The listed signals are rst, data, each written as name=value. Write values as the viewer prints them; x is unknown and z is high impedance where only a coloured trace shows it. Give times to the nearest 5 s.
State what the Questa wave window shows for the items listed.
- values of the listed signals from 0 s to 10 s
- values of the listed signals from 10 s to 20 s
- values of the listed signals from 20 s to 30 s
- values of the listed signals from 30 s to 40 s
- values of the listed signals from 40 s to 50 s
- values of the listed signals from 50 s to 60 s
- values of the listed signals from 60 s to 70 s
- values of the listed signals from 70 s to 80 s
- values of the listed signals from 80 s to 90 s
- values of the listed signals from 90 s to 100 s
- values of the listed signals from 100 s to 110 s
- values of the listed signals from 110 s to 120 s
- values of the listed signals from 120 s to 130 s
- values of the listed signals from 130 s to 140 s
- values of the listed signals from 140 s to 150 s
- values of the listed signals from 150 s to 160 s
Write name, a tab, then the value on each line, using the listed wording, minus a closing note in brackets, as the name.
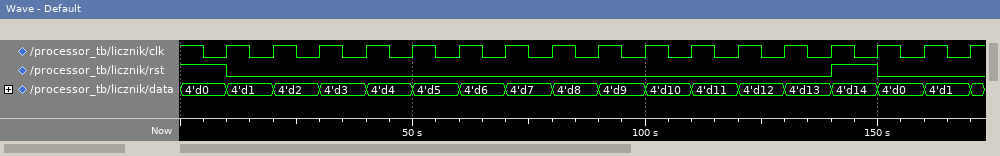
values of the listed signals from 0 s to 10 s	rst=1, data=4'd0
values of the listed signals from 10 s to 20 s	rst=0, data=4'd1
values of the listed signals from 20 s to 30 s	rst=0, data=4'd2
values of the listed signals from 30 s to 40 s	rst=0, data=4'd3
values of the listed signals from 40 s to 50 s	rst=0, data=4'd4
values of the listed signals from 50 s to 60 s	rst=0, data=4'd5
values of the listed signals from 60 s to 70 s	rst=0, data=4'd6
values of the listed signals from 70 s to 80 s	rst=0, data=4'd7
values of the listed signals from 80 s to 90 s	rst=0, data=4'd8
values of the listed signals from 90 s to 100 s	rst=0, data=4'd9
values of the listed signals from 100 s to 110 s	rst=0, data=4'd10
values of the listed signals from 110 s to 120 s	rst=0, data=4'd11
values of the listed signals from 120 s to 130 s	rst=0, data=4'd12
values of the listed signals from 130 s to 140 s	rst=0, data=4'd13
values of the listed signals from 140 s to 150 s	rst=1, data=4'd14
values of the listed signals from 150 s to 160 s	rst=0, data=4'd0
